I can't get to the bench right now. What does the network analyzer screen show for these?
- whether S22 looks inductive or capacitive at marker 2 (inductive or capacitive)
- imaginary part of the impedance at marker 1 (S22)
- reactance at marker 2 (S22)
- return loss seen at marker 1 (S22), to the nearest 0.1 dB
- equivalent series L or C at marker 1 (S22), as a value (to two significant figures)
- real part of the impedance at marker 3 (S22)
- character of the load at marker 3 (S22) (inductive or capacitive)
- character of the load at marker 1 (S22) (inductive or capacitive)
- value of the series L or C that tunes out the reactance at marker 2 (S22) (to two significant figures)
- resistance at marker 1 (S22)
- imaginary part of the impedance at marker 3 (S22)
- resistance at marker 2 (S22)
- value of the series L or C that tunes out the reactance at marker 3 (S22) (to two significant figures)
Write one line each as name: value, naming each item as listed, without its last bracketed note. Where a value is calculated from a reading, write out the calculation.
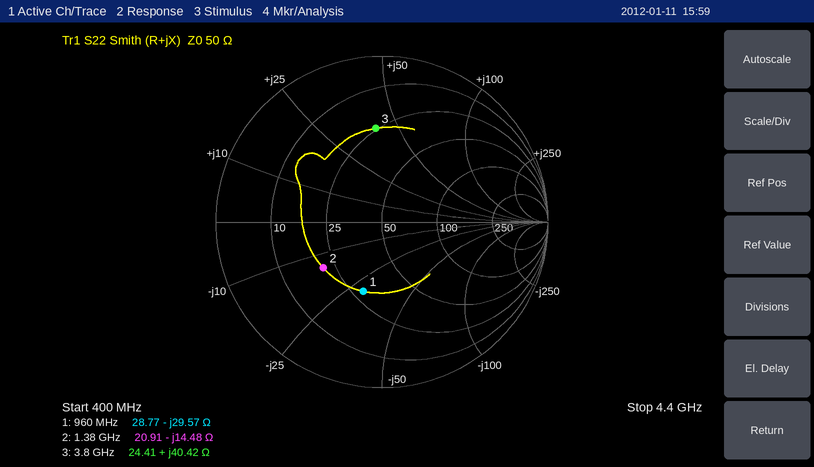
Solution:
whether S22 looks inductive or capacitive at marker 2: capacitive
imaginary part of the impedance at marker 1: -29.57 Ω
reactance at marker 2: -14.48 Ω
return loss seen at marker 1 (S22), to the nearest 0.1 dB: 7.3 dB
equivalent series L or C at marker 1 (S22), as a value: C = 1/(2π × 960 MHz × 29.57 Ω) ≈ 5.6 pF
real part of the impedance at marker 3: 24.41 Ω
character of the load at marker 3 (S22): inductive
character of the load at marker 1 (S22): capacitive
value of the series L or C that tunes out the reactance at marker 2 (S22): L = 14.48 Ω/(2π × 1.38 GHz) ≈ 1.7 nH
resistance at marker 1: 28.77 Ω
imaginary part of the impedance at marker 3: +40.42 Ω
resistance at marker 2: 20.91 Ω
value of the series L or C that tunes out the reactance at marker 3 (S22): C = 1/(2π × 3.8 GHz × 40.42 Ω) ≈ 1.0 pF
